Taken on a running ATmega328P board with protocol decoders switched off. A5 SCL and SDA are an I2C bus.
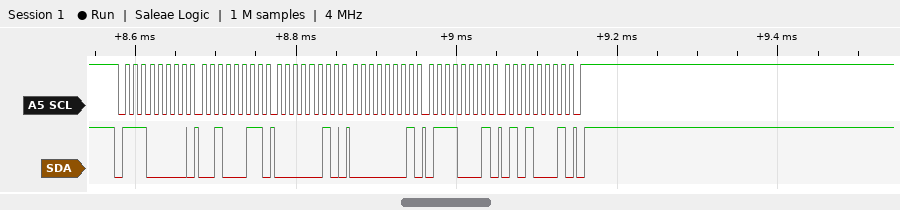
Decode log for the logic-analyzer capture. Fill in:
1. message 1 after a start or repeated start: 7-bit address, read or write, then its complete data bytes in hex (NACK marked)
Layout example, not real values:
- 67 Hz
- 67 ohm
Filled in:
- 0x70 write: 23 02 01 71 51
